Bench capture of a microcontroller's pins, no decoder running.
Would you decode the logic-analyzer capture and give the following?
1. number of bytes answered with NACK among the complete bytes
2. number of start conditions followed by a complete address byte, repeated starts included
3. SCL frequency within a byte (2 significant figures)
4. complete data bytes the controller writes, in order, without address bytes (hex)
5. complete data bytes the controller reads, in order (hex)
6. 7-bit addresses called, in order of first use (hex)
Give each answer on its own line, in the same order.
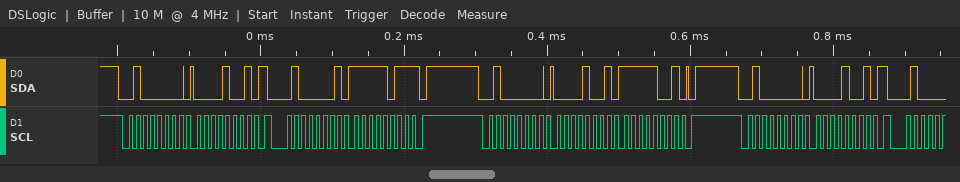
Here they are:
1
4
100 kHz
09 09 F9 09
FB
0x20
